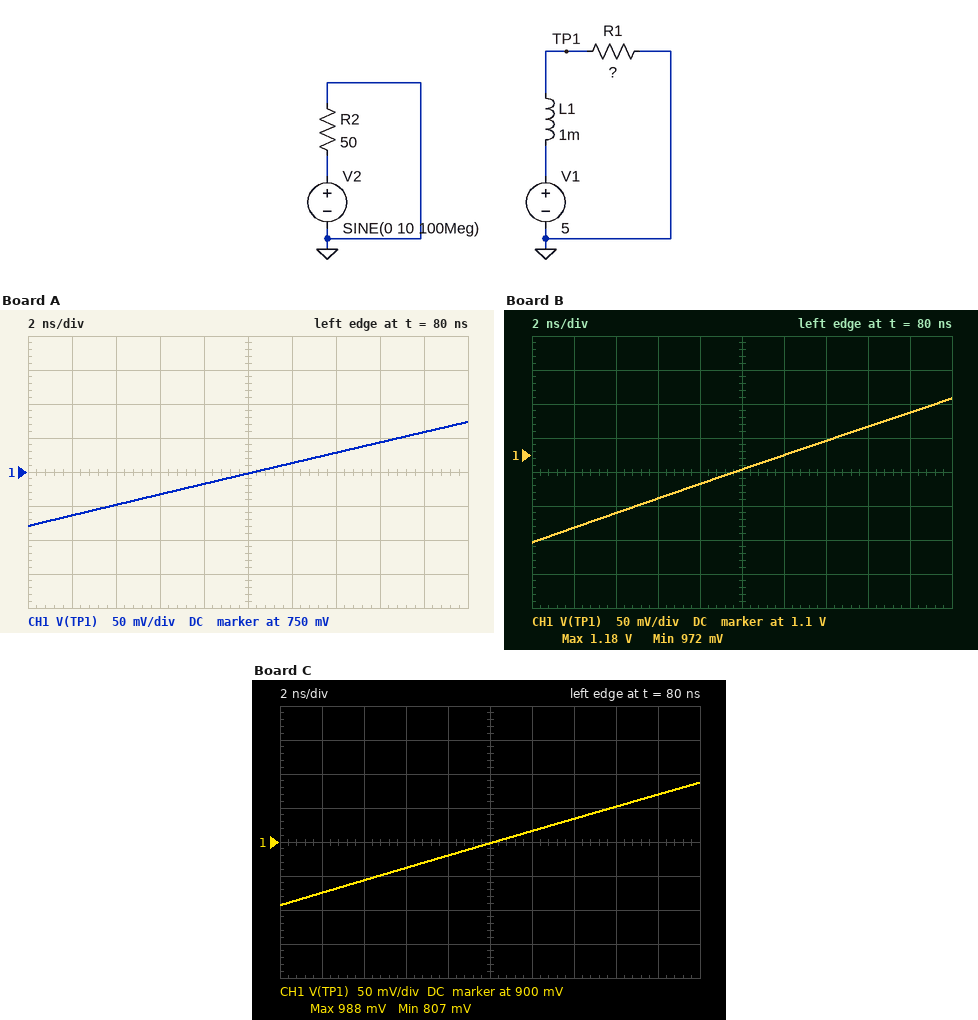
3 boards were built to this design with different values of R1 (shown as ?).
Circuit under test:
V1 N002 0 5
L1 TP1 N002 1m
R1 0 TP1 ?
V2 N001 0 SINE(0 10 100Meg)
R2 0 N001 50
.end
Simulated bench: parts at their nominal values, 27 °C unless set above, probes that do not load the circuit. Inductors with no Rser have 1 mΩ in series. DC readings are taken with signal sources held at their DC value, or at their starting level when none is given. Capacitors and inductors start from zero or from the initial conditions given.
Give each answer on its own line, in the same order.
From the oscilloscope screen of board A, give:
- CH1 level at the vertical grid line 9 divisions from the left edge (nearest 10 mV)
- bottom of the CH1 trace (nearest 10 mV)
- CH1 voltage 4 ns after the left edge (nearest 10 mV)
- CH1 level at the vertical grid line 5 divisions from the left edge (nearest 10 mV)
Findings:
810 mV
670 mV
700 mV
750 mV
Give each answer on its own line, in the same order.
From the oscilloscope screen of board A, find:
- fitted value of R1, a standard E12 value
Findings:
1.8 kΩ
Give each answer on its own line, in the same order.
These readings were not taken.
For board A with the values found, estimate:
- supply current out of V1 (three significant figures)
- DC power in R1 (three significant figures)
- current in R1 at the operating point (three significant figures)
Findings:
2.78 mA
13.9 mW
2.78 mA
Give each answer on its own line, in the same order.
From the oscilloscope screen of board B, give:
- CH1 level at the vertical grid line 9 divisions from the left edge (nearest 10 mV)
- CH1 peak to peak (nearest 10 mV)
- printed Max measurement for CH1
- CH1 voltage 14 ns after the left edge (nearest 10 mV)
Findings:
1.16 V
210 mV
1.18 V
1.12 V
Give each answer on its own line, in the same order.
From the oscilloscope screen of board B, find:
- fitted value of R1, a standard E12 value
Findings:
2.7 kΩ
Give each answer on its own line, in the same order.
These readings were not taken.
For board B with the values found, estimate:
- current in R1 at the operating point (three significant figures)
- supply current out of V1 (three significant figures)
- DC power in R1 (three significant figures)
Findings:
1.85 mA
1.85 mA
9.26 mW
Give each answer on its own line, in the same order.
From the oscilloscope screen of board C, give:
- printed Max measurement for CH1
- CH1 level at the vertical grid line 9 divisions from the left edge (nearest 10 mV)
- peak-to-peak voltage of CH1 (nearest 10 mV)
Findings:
988 mV
970 mV
180 mV
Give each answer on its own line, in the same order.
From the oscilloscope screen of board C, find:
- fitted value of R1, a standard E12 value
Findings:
2.2 kΩ
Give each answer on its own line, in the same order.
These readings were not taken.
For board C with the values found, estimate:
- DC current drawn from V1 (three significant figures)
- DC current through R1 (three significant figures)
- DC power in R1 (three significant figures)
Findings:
2.27 mA
2.27 mA
11.4 mW
